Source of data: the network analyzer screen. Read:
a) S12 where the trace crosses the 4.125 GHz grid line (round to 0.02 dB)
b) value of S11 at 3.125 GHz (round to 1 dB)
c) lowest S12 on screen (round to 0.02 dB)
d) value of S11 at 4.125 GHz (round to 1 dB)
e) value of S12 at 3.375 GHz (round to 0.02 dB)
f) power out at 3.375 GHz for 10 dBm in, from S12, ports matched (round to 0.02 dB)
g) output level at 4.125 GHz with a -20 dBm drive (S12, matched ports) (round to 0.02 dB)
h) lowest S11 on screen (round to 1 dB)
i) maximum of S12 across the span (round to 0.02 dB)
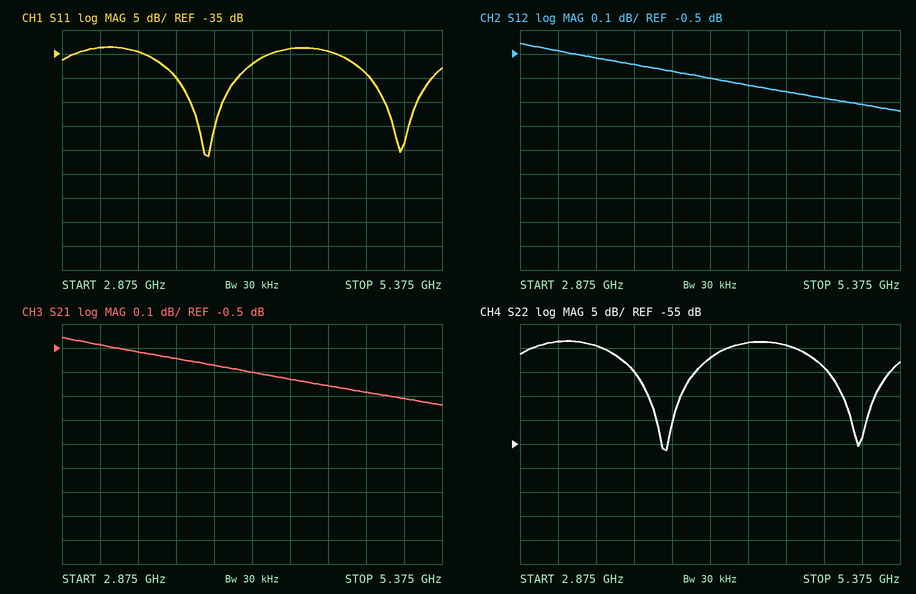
-0.60 dB
-34 dB
-0.74 dB
-37 dB
-0.52 dB
9.48 dBm
-20.60 dBm
-56 dB
-0.46 dB
